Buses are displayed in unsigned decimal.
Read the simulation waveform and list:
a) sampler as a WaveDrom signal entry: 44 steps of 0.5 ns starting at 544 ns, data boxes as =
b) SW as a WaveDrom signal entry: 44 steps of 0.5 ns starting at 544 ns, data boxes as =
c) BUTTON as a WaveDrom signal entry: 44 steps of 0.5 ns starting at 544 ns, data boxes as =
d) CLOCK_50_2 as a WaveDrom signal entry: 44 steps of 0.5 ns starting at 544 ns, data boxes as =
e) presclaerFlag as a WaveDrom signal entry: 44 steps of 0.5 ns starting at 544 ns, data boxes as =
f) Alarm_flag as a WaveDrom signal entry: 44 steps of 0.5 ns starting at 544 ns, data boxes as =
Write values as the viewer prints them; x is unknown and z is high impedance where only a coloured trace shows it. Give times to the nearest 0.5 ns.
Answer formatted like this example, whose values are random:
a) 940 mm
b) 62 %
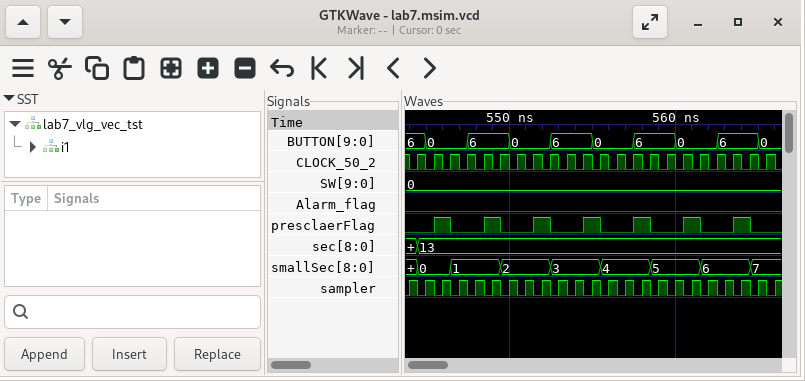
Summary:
a) {name: 'sampler', wave: '10101010101010101010101010101010101010101010'}
b) {name: 'SW', wave: '=...........................................', data: '0'}
c) {name: 'BUTTON', wave: '=.=....=....=....=....=....=....=....=....=.', data: '6 0 6 0 6 0 6 0 6 0'}
d) {name: 'CLOCK_50_2', wave: '01010101010101010101010101010101010101010101'}
e) {name: 'presclaerFlag', wave: '0..1.0...1.0...1.0...1.0...1.0...1.0...1.0..'}
f) {name: 'Alarm_flag', wave: '0...........................................'}
